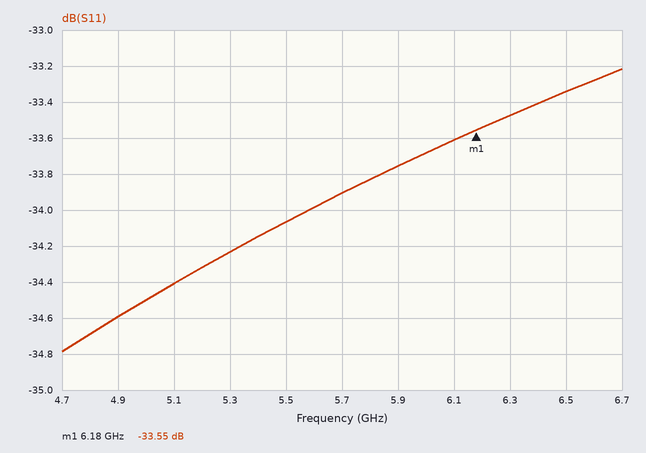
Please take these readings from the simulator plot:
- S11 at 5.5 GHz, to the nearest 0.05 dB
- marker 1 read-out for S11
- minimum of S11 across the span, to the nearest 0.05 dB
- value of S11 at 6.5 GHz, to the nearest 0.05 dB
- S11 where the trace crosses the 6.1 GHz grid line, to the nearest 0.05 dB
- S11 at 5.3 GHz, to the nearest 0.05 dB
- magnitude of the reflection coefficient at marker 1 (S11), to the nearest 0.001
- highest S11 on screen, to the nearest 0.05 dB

-34.05 dB
-33.55 dB
-34.80 dB
-33.35 dB
-33.60 dB
-34.25 dB
0.021
-33.20 dB
